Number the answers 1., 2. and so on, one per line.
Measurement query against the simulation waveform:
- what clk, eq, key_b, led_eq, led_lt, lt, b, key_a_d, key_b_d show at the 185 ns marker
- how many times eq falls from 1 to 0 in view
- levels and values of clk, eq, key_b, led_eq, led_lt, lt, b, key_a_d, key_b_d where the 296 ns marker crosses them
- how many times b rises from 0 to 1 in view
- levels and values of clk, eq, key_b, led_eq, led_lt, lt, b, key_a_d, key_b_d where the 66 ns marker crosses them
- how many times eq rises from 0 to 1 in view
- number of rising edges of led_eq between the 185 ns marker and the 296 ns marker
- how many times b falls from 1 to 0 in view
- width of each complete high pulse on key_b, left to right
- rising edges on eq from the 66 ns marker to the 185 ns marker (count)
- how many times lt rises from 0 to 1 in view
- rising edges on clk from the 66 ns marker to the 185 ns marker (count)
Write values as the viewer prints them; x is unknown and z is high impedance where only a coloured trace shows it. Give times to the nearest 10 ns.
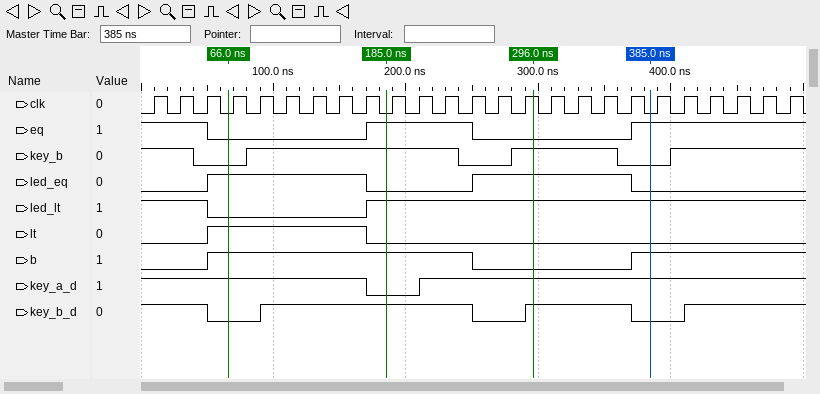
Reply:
1. clk=0, eq=1, key_b=1, led_eq=0, led_lt=1, lt=0, b=1, key_a_d=0, key_b_d=1
2. 2
3. clk=1, eq=0, key_b=1, led_eq=1, led_lt=1, lt=0, b=0, key_a_d=1, key_b_d=1
4. 2
5. clk=0, eq=0, key_b=0, led_eq=1, led_lt=0, lt=1, b=1, key_a_d=1, key_b_d=0
6. 2
7. 1
8. 1
9. 160 ns, 80 ns
10. 1
11. 1
12. 6
